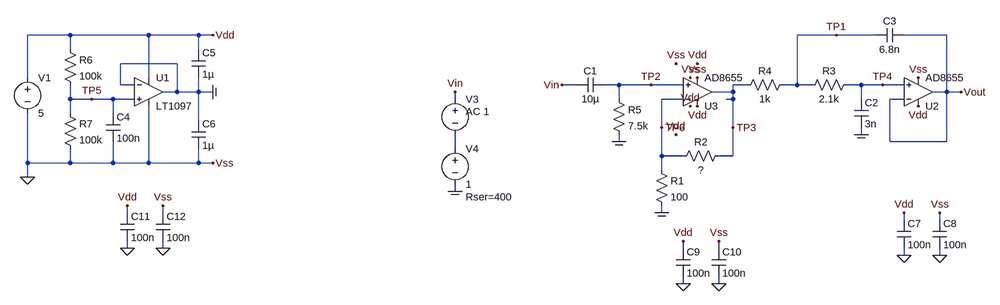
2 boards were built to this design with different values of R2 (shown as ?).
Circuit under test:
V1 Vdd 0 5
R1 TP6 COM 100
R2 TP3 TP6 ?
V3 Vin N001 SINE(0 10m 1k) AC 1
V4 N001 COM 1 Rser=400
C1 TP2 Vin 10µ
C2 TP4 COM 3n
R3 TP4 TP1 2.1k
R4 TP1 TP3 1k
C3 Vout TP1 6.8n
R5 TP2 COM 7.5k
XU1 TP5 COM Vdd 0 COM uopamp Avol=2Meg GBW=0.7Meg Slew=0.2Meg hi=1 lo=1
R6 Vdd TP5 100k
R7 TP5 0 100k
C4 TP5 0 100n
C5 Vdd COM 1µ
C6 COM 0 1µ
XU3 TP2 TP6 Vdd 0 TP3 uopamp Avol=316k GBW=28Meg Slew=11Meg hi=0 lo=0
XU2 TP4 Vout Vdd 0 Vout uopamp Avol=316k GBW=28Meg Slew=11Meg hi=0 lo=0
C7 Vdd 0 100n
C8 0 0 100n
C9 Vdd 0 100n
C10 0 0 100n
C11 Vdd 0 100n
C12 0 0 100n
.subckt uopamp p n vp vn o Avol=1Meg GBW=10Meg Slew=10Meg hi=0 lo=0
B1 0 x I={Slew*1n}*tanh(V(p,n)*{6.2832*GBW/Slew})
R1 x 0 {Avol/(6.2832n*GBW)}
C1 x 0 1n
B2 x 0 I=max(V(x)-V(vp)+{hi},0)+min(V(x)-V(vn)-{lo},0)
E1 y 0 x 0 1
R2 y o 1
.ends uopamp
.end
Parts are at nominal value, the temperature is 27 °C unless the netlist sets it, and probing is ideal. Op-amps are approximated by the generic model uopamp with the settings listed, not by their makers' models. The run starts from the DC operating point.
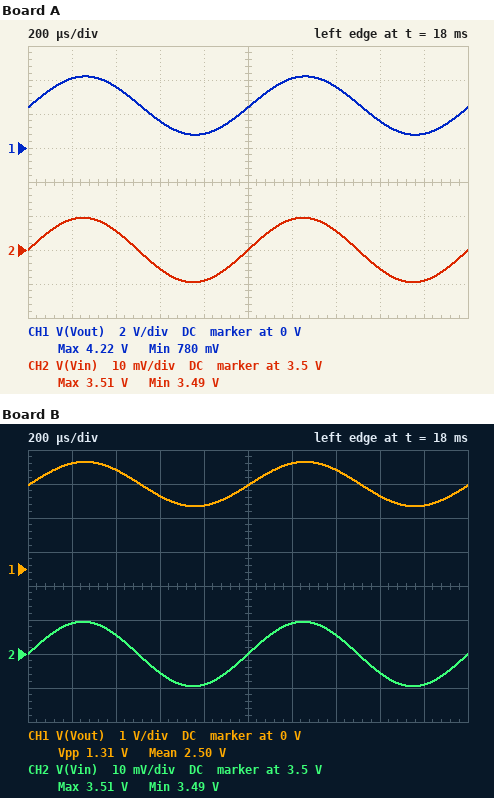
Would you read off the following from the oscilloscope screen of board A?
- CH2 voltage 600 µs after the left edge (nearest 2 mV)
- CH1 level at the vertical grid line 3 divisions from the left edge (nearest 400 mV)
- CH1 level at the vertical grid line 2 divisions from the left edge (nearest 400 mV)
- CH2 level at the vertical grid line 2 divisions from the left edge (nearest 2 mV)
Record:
3.494 V
1.6 V
3.6 V
3.506 V
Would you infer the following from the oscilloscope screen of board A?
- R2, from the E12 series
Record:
18 kΩ
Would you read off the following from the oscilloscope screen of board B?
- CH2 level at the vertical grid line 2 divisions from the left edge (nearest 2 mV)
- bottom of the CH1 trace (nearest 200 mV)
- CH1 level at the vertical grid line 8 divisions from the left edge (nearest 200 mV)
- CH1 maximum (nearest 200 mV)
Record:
3.506 V
1.8 V
2.2 V
3.2 V
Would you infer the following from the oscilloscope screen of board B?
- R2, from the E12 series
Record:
6.8 kΩ
